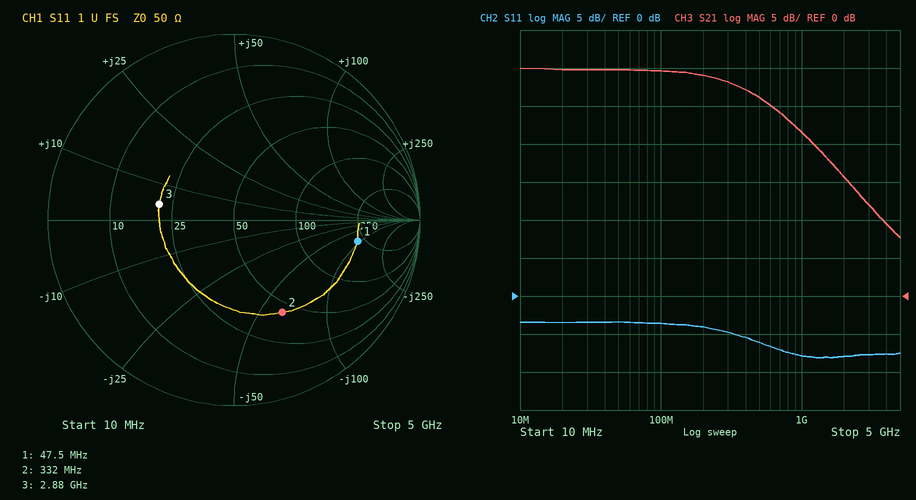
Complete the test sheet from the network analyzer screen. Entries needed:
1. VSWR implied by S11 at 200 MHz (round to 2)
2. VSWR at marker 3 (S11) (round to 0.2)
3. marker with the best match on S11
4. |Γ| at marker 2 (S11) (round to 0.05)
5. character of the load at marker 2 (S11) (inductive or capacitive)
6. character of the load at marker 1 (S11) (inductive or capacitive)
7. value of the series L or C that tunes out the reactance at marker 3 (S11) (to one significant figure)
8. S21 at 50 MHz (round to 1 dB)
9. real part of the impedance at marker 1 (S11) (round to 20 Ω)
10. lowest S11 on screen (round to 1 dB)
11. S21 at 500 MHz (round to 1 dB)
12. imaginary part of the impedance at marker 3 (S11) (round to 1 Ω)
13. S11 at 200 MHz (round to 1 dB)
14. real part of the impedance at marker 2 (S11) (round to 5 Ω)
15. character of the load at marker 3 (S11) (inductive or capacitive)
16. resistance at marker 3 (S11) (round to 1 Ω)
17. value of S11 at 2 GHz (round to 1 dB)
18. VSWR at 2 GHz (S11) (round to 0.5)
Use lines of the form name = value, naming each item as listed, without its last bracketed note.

VSWR implied by S11 at 200 MHz = 4
VSWR at marker 3 (S11) = 2.4
marker with the best match on S11 = marker 3
|Γ| at marker 2 (S11) = 0.55
character of the load at marker 2 (S11) = capacitive
character of the load at marker 1 (S11) = capacitive
value of the series L or C that tunes out the reactance at marker 3 (S11) = 10 pF
S21 at 50 MHz = 30 dB
real part of the impedance at marker 1 (S11) = 220 Ω
lowest S11 on screen = -8 dB
S21 at 500 MHz = 26 dB
imaginary part of the impedance at marker 3 (S11) = +4 Ω
S11 at 200 MHz = -4 dB
real part of the impedance at marker 2 (S11) = 45 Ω
character of the load at marker 3 (S11) = inductive
resistance at marker 3 (S11) = 21 Ω
value of S11 at 2 GHz = -8 dB
VSWR at 2 GHz (S11) = 2.5
